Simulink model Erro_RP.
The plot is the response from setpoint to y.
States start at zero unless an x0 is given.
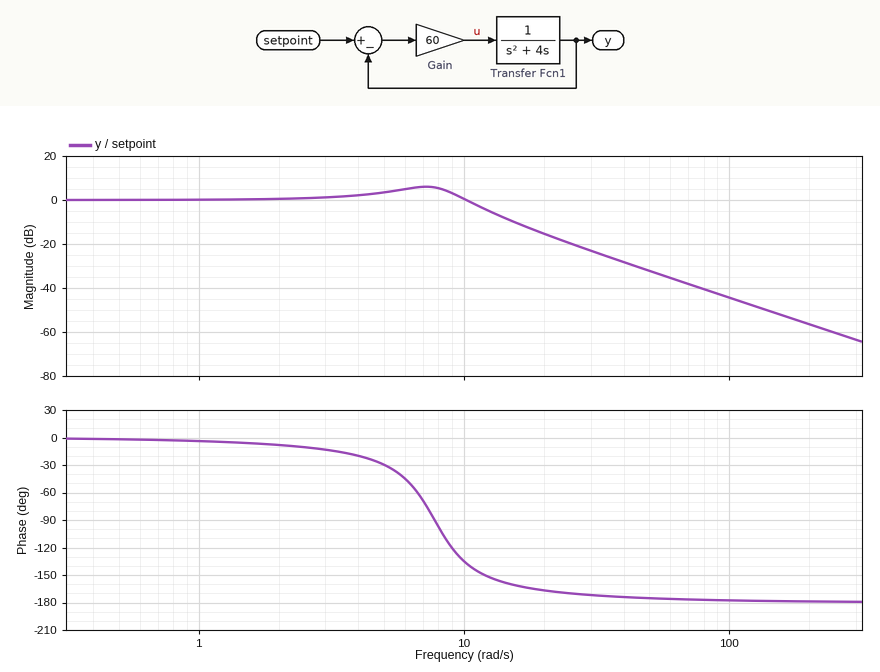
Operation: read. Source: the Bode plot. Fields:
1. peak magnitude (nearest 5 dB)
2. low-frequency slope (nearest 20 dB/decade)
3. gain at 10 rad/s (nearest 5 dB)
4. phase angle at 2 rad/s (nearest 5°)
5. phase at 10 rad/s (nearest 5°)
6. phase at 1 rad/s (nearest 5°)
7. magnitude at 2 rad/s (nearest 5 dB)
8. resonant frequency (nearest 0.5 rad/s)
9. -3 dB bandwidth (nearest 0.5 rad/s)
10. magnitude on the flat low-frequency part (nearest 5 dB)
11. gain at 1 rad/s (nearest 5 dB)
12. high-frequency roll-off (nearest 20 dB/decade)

5 dB
0 dB/decade
0 dB
-10°
-135°
-5°
0 dB
7.0 rad/s
11.5 rad/s
0 dB
0 dB
-40 dB/decade
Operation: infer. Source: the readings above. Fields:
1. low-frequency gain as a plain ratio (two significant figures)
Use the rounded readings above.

1.0
